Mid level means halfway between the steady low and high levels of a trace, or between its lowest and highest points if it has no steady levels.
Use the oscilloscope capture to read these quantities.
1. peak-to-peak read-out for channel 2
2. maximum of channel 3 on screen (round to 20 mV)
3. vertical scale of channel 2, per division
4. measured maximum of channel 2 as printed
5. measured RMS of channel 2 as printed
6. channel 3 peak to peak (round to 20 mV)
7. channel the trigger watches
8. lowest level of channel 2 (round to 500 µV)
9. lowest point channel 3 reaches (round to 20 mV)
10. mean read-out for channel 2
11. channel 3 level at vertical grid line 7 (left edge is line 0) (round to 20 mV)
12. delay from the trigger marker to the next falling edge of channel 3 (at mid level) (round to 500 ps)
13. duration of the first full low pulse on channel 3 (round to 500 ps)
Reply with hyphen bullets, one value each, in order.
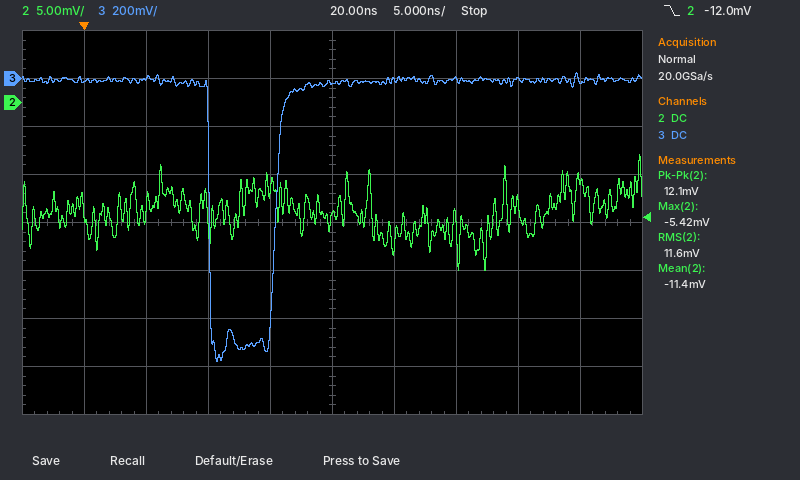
- 12.1 mV
- 20 mV
- 5 mV
- -5.42 mV
- 11.6 mV
- 1.20 V
- channel 2
- -17.5 mV
- -1.18 V
- -11.4 mV
- 0 mV
- 10.0 ns
- 5.5 ns
